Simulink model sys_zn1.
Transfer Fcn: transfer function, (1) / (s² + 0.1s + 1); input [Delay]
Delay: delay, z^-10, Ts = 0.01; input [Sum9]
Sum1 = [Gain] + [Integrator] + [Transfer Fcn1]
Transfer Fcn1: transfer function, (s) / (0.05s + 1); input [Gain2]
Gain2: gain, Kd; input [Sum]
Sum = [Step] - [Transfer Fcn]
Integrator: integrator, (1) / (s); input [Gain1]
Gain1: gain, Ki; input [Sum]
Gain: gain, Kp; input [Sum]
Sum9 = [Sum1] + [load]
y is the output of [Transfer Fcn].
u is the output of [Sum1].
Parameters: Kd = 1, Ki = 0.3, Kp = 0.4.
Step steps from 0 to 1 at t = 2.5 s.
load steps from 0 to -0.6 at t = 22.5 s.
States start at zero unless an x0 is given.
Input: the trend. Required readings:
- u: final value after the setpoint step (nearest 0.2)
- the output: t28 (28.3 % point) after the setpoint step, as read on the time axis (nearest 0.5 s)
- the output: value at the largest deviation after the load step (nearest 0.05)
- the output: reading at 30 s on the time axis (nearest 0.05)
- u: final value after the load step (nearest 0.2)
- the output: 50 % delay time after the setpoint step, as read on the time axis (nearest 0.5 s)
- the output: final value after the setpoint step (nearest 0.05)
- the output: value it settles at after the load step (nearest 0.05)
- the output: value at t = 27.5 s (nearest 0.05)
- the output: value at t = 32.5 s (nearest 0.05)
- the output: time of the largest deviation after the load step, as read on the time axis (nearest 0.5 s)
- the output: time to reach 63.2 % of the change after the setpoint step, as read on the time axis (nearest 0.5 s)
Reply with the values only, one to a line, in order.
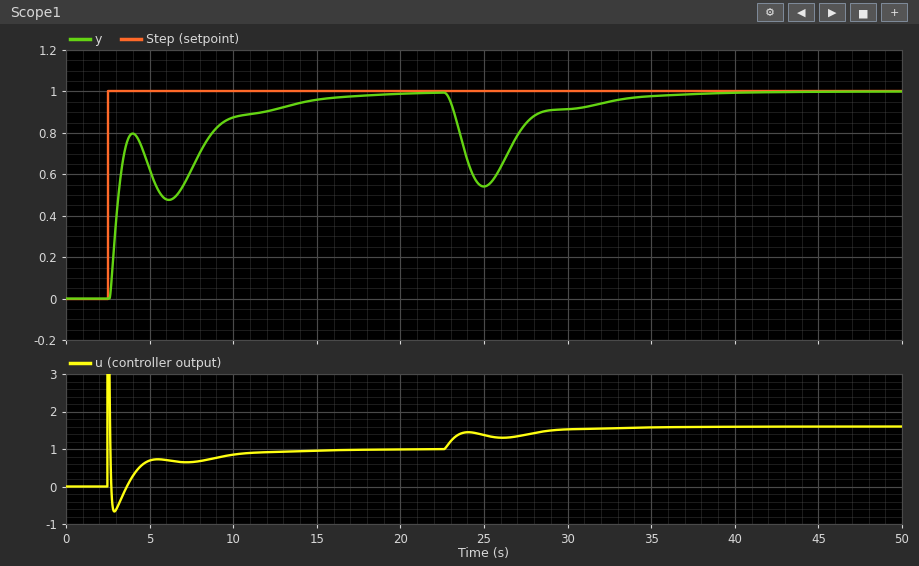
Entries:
1.0
3.0 s
0.55
0.90
1.6
3.0 s
1.00
1.00
0.85
0.95
25.0 s
3.5 s
